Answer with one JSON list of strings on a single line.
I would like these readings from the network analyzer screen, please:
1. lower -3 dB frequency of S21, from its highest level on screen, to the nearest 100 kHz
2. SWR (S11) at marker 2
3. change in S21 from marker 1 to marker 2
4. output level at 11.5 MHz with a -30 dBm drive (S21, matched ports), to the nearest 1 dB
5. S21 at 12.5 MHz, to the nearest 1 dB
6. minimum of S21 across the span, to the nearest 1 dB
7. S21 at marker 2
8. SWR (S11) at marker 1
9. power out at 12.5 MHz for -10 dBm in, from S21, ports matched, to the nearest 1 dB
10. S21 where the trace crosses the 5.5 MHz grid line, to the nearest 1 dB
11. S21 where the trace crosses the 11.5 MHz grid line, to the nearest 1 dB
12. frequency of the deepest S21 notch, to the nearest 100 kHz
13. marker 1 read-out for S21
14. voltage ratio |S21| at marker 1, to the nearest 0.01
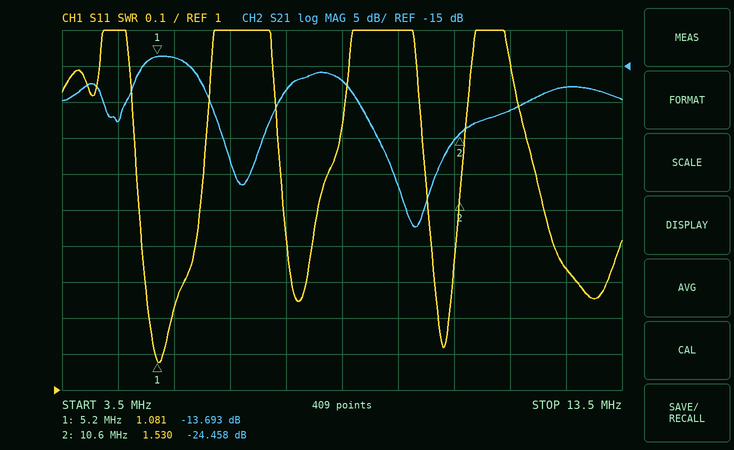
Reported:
["4.8 MHz", "1.530", "-10.765 dB", "-51 dBm", "-18 dB", "-37 dB", "-24.458 dB", "1.081", "-28 dBm", "-14 dB", "-21 dB", "9.8 MHz", "-13.693 dB", "0.21"]
